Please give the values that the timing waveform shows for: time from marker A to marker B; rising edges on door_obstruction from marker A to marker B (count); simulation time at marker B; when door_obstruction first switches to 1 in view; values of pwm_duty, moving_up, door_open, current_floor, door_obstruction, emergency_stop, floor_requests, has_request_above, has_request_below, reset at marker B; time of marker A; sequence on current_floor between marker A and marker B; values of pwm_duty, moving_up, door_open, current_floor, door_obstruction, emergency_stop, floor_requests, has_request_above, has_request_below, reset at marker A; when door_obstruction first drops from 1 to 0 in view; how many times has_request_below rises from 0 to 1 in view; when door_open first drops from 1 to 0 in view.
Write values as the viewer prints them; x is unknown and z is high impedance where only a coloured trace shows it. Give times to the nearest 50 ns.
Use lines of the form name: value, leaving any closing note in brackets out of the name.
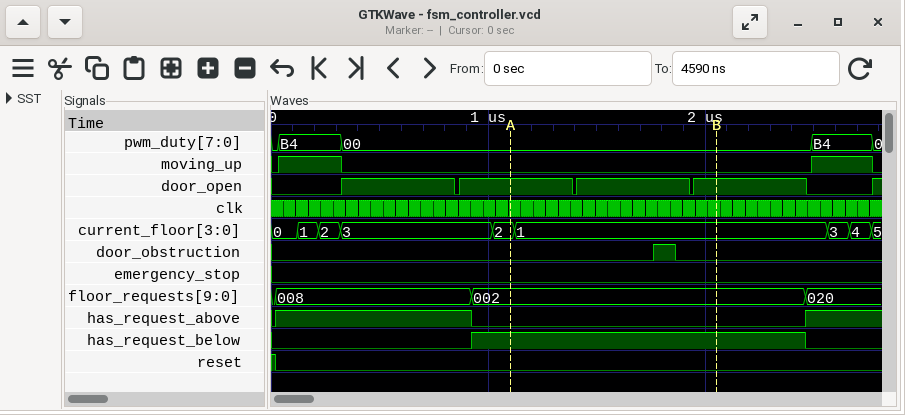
time from marker A to marker B: 950 ns
rising edges on door_obstruction from marker A to marker B: 1
simulation time at marker B: 2050 ns
when door_obstruction first switches to 1 in view: 1750 ns
values of pwm_duty, moving_up, door_open, current_floor, door_obstruction, emergency_stop, floor_requests, has_request_above, has_request_below, reset at marker B: pwm_duty=00, moving_up=0, door_open=1, current_floor=1, door_obstruction=0, emergency_stop=0, floor_requests=002, has_request_above=0, has_request_below=1, reset=0
time of marker A: 1100 ns
sequence on current_floor between marker A and marker B: 2, 1
values of pwm_duty, moving_up, door_open, current_floor, door_obstruction, emergency_stop, floor_requests, has_request_above, has_request_below, reset at marker A: pwm_duty=00, moving_up=0, door_open=1, current_floor=2, door_obstruction=0, emergency_stop=0, floor_requests=002, has_request_above=0, has_request_below=1, reset=0
when door_obstruction first drops from 1 to 0 in view: 1850 ns
how many times has_request_below rises from 0 to 1 in view: 1
when door_open first drops from 1 to 0 in view: 850 ns
